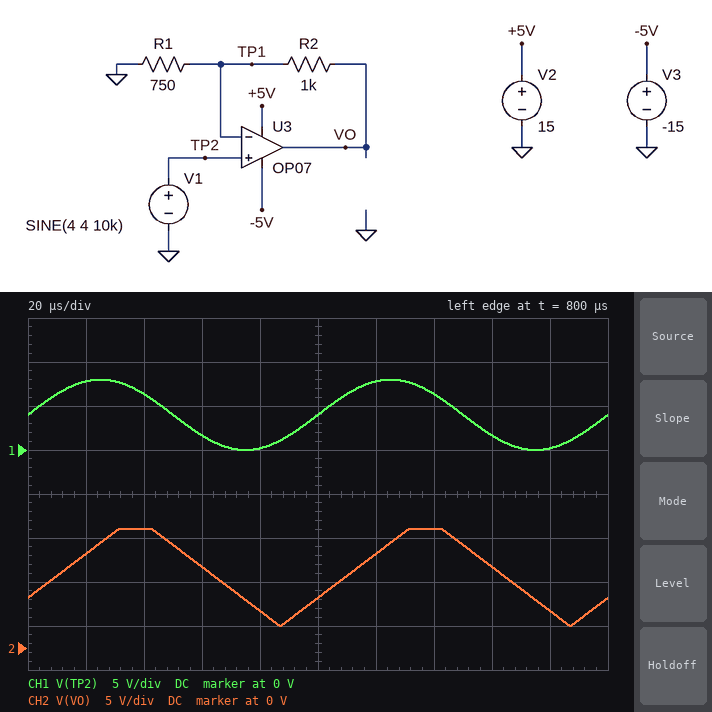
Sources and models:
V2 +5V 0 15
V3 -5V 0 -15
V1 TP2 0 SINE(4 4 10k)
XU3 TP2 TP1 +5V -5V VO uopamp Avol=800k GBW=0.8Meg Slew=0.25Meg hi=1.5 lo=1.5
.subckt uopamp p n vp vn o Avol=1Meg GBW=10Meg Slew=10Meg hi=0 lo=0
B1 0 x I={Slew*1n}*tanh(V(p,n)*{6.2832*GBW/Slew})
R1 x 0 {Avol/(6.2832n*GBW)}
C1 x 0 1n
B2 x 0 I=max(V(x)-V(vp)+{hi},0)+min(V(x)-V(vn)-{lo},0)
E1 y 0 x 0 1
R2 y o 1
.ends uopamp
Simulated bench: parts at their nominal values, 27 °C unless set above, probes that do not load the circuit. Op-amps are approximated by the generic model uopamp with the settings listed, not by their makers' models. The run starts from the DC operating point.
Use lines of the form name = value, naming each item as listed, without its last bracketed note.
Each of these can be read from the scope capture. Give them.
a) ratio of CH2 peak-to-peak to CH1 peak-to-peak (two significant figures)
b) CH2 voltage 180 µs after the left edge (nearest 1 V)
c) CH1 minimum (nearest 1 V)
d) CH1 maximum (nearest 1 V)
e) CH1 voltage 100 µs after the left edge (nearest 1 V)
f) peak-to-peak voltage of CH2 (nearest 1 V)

ratio of CH2 peak-to-peak to CH1 peak-to-peak = 1.4
CH2 voltage 180 µs after the left edge = 4 V
CH1 minimum = 0 V
CH1 maximum = 8 V
CH1 voltage 100 µs after the left edge = 4 V
peak-to-peak voltage of CH2 = 11 V
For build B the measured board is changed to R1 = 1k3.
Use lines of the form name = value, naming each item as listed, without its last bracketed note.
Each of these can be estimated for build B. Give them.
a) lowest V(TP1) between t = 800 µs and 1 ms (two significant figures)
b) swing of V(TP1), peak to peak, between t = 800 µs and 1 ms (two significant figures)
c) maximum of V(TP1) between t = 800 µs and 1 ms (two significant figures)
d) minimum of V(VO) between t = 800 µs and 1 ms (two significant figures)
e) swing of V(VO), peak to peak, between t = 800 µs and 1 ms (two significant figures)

lowest V(TP1) between t = 800 µs and 1 ms = 530 mV
swing of V(TP1), peak to peak, between t = 800 µs and 1 ms = 6.9 V
maximum of V(TP1) between t = 800 µs and 1 ms = 7.5 V
minimum of V(VO) between t = 800 µs and 1 ms = 940 mV
swing of V(VO), peak to peak, between t = 800 µs and 1 ms = 12 V
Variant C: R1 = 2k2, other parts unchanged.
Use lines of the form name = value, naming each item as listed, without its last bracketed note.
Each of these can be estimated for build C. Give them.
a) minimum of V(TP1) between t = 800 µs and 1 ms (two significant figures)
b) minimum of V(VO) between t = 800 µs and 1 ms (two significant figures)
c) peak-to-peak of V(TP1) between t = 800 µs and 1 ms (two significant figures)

minimum of V(TP1) between t = 800 µs and 1 ms = 62 mV
minimum of V(VO) between t = 800 µs and 1 ms = 90 mV
peak-to-peak of V(TP1) between t = 800 µs and 1 ms = 7.9 V
